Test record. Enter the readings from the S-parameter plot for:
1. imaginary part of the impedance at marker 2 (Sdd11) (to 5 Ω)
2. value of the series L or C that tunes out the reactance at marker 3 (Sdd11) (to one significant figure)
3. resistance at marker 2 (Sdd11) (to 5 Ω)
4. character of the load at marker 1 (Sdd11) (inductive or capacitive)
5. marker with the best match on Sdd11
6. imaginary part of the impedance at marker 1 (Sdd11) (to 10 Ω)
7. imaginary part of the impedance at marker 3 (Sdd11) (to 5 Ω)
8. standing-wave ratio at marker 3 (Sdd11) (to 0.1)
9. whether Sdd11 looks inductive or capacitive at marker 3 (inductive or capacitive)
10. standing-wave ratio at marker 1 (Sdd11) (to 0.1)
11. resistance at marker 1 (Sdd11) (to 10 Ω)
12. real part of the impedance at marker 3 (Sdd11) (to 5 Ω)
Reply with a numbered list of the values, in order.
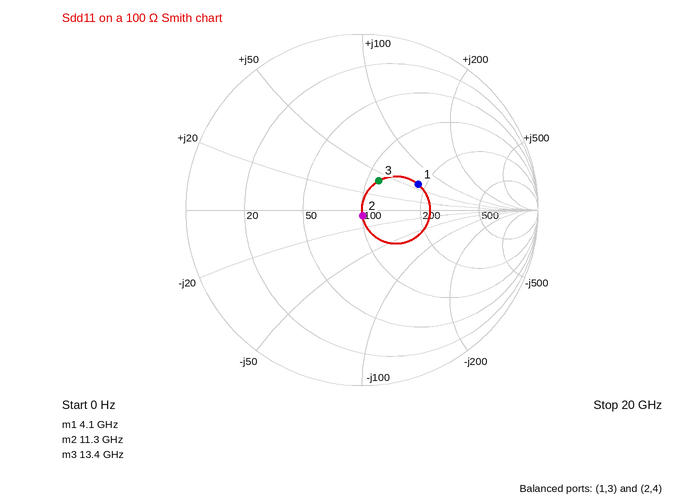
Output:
1. -5 Ω
2. 300 fF
3. 100 Ω
4. inductive
5. marker 2
6. +60 Ω
7. +40 Ω
8. 1.5
9. inductive
10. 2.1
11. 180 Ω
12. 115 Ω
